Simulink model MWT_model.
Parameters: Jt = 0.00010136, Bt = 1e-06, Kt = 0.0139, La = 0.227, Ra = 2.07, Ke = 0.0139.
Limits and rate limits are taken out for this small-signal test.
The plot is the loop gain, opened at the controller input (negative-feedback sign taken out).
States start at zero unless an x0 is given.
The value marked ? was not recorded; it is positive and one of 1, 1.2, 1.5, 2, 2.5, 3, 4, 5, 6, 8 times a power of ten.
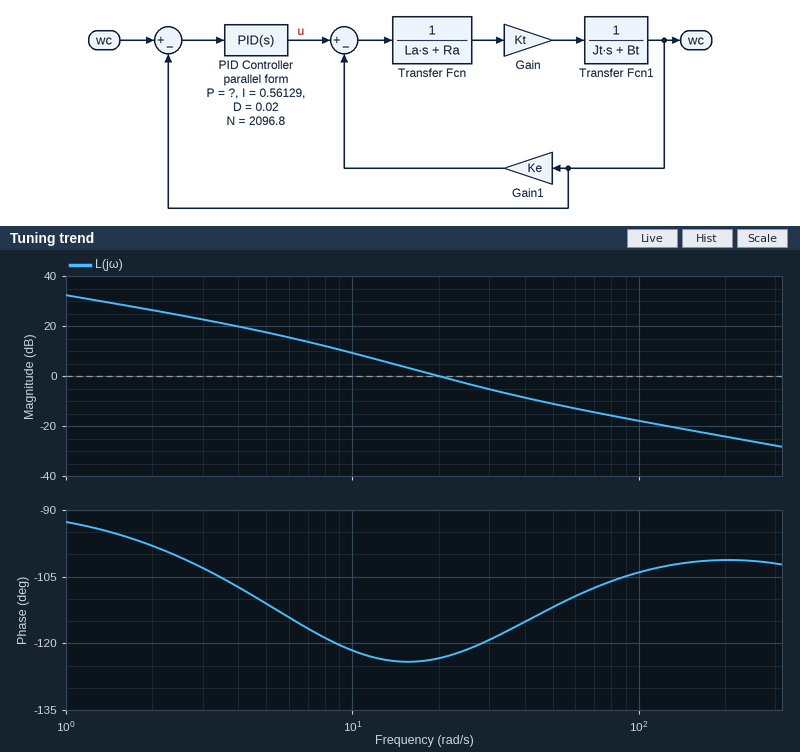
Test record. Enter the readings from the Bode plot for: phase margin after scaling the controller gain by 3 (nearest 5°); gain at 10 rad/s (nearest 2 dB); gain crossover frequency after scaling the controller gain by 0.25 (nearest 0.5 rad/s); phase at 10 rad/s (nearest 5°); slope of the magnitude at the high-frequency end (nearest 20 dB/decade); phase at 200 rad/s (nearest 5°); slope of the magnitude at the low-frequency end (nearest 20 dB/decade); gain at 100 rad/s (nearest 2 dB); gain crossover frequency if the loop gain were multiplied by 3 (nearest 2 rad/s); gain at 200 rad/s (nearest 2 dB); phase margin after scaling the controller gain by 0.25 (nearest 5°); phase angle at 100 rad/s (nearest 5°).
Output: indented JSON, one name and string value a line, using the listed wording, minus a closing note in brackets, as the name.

{
  "phase margin after scaling the controller gain by 3": "65°",
  "gain at 10 rad/s": "10 dB",
  "gain crossover frequency after scaling the controller gain by 0.25": "8.0 rad/s",
  "phase at 10 rad/s": "-120°",
  "slope of the magnitude at the high-frequency end": "-20 dB/decade",
  "phase at 200 rad/s": "-100°",
  "slope of the magnitude at the low-frequency end": "-20 dB/decade",
  "gain at 100 rad/s": "-18 dB",
  "gain crossover frequency if the loop gain were multiplied by 3": "44 rad/s",
  "gain at 200 rad/s": "-24 dB",
  "phase margin after scaling the controller gain by 0.25": "60°",
  "phase angle at 100 rad/s": "-105°"
}
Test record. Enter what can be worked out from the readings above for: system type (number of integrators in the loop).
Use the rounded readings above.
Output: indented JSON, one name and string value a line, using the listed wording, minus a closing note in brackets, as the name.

{
  "system type": "1"
}
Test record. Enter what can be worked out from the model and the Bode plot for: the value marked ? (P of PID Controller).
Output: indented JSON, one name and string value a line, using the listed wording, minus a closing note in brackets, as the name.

{
  "the value marked ?": "0.6"
}
